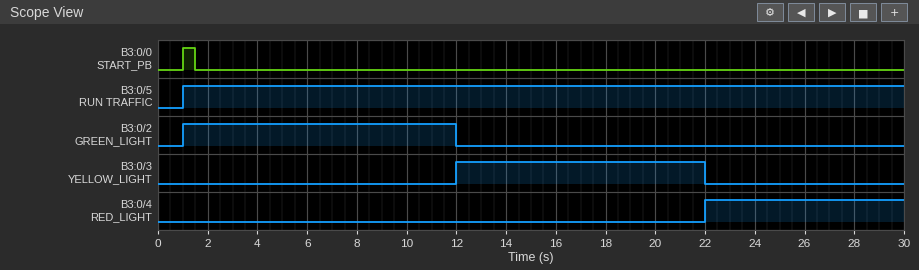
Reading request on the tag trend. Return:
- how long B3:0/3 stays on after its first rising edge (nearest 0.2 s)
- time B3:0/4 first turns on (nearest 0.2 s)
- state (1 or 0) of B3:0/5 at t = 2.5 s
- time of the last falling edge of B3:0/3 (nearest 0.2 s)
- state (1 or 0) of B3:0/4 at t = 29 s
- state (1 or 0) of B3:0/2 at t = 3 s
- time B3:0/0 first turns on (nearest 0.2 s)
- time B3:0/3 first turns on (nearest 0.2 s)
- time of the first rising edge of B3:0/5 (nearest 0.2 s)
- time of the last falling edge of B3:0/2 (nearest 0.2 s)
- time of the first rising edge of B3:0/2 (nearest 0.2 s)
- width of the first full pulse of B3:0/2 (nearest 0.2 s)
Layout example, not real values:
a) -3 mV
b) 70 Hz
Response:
a) 10.0 s
b) 22.0 s
c) 1
d) 22.0 s
e) 1
f) 1
g) 1.0 s
h) 12.0 s
i) 1.0 s
j) 12.0 s
k) 1.0 s
l) 11.0 s
